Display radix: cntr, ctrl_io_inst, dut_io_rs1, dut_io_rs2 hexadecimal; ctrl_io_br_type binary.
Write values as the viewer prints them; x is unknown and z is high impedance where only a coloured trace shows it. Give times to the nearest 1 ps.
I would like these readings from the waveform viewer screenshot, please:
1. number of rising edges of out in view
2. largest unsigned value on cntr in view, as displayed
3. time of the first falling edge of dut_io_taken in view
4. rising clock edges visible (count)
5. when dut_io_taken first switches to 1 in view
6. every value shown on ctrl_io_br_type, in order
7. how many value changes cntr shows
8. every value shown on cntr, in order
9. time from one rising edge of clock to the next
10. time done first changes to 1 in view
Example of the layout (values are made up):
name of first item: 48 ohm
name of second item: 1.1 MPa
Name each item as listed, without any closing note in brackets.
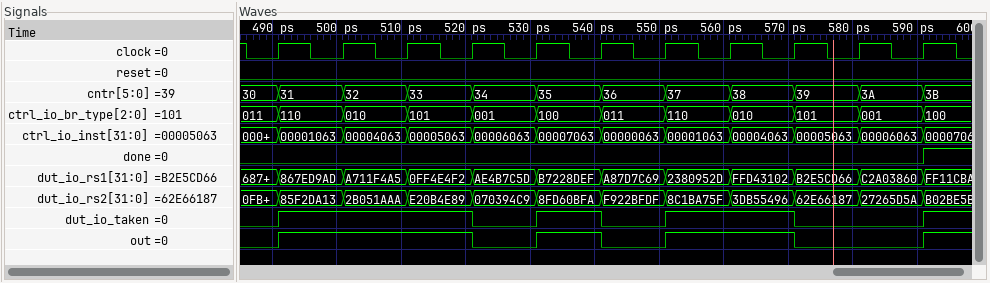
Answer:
number of rising edges of out in view: 4
largest unsigned value on cntr in view, as displayed: 3B
time of the first falling edge of dut_io_taken in view: 521 ps
rising clock edges visible: 11
when dut_io_taken first switches to 1 in view: 491 ps
every value shown on ctrl_io_br_type, in order: 011, 110, 010, 101, 001, 100, 011, 110, 010, 101, 001, 100
how many value changes cntr shows: 11
every value shown on cntr, in order: 30, 31, 32, 33, 34, 35, 36, 37, 38, 39, 3A, 3B
time from one rising edge of clock to the next: 10 ps
time done first changes to 1 in view: 591 ps
